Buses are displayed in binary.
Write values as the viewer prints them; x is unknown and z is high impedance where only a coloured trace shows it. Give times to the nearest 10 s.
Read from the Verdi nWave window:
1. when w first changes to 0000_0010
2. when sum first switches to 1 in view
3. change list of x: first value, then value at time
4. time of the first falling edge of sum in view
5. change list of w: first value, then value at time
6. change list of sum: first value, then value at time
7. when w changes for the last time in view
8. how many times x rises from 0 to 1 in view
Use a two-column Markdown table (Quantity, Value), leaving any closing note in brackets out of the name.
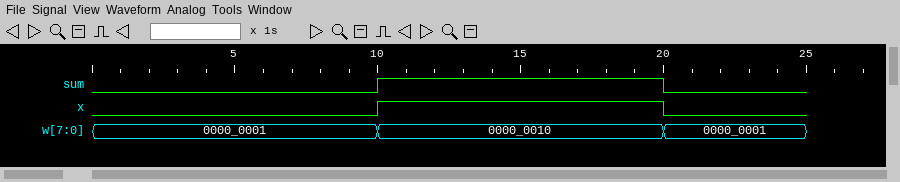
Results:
| Quantity | Value |
|---|---|
| when w first changes to 0000_0010 | 10 s |
| when sum first switches to 1 in view | 10 s |
| change list of x: first value, then value at time | 0, 1 at 10 s, 0 at 20 s |
| time of the first falling edge of sum in view | 20 s |
| change list of w: first value, then value at time | 0000_0001, 0000_0010 at 10 s, 0000_0001 at 20 s |
| change list of sum: first value, then value at time | 0, 1 at 10 s, 0 at 20 s |
| when w changes for the last time in view | 20 s |
| how many times x rises from 0 to 1 in view | 1 |
